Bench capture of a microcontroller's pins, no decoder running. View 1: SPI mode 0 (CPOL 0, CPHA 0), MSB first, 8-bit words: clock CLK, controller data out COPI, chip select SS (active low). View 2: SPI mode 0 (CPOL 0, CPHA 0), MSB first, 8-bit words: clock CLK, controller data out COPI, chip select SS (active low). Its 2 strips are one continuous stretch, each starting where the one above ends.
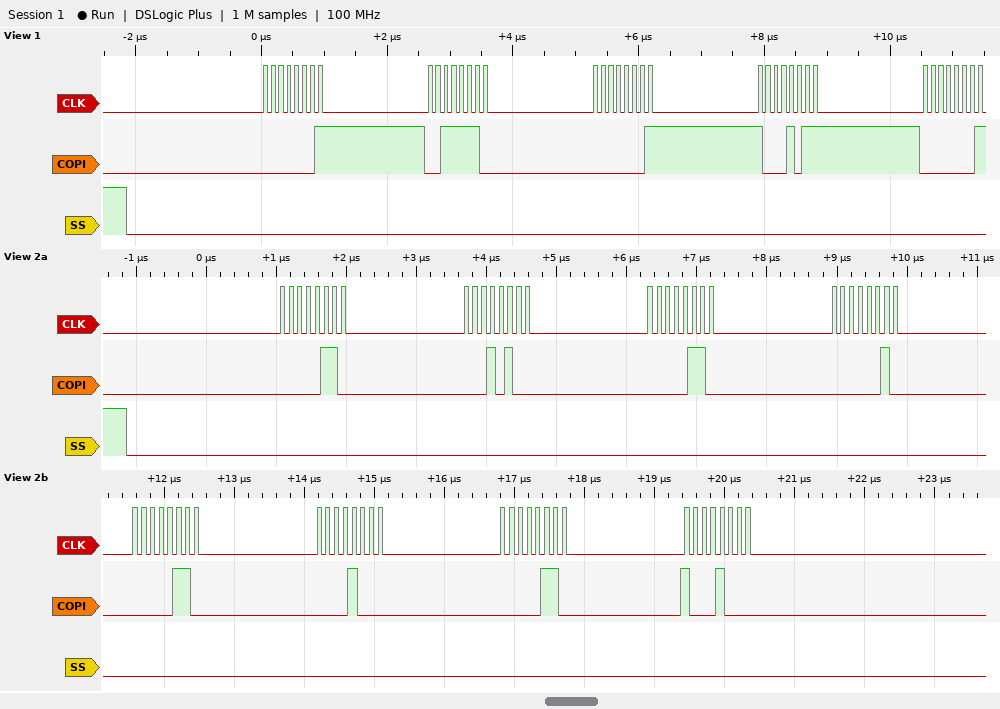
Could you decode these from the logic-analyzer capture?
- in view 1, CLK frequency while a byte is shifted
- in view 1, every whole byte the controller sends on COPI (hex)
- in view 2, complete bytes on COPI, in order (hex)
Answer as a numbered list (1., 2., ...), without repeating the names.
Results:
1. 8 MHz
2. 01 3E 01 8B 01
3. 0x06 0x14 0x06 0x02 0x06 0x08 0x06 0x88
